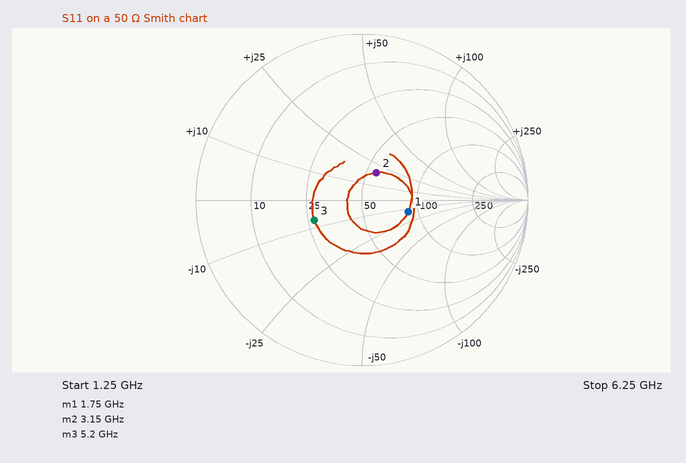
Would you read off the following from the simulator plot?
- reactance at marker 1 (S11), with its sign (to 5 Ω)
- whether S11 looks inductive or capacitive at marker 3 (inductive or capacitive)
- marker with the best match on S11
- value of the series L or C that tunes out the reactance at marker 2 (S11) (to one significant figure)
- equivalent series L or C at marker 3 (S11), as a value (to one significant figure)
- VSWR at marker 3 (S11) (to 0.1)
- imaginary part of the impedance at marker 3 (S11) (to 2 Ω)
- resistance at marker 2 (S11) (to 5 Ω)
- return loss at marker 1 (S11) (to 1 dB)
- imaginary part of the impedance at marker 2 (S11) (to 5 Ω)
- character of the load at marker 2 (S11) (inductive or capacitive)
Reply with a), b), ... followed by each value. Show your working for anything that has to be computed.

a) -15 Ω
b) capacitive
c) marker 2
d) C = 1/(2π × 3.15 GHz × 20 Ω) ≈ 3 pF
e) C = 1/(2π × 5.2 GHz × 8 Ω) ≈ 4 pF
f) 1.9
g) -8 Ω
h) 55 Ω
i) 11 dB
j) +20 Ω
k) inductive
